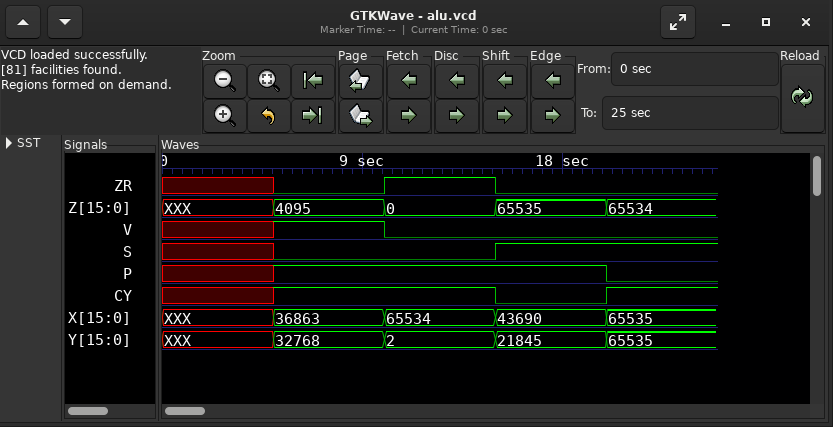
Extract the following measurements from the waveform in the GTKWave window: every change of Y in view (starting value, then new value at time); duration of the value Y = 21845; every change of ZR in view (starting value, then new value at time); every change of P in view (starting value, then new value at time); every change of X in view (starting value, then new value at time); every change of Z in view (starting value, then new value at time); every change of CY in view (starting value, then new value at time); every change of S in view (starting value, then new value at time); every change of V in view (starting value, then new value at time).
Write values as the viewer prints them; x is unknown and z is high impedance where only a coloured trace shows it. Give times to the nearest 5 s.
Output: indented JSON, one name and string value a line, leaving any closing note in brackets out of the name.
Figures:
{
  "every change of Y in view": "XXX, 32768 at 5 s, 2 at 10 s, 21845 at 15 s, 65535 at 20 s",
  "duration of the value Y = 21845": "5 s",
  "every change of ZR in view": "x, 0 at 5 s, 1 at 10 s, 0 at 15 s",
  "every change of P in view": "x, 1 at 5 s, 0 at 20 s",
  "every change of X in view": "XXX, 36863 at 5 s, 65534 at 10 s, 43690 at 15 s, 65535 at 20 s",
  "every change of Z in view": "XXX, 4095 at 5 s, 0 at 10 s, 65535 at 15 s, 65534 at 20 s",
  "every change of CY in view": "x, 1 at 5 s, 0 at 15 s, 1 at 20 s",
  "every change of S in view": "x, 0 at 5 s, 1 at 15 s",
  "every change of V in view": "x, 1 at 5 s, 0 at 10 s"
}
